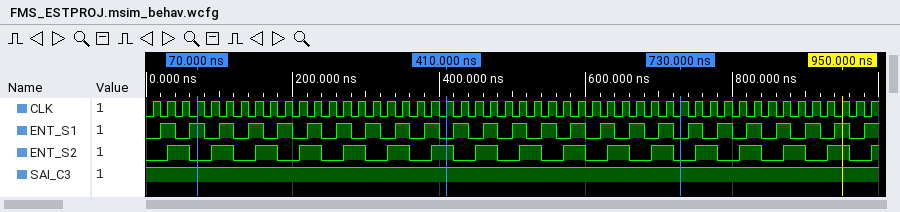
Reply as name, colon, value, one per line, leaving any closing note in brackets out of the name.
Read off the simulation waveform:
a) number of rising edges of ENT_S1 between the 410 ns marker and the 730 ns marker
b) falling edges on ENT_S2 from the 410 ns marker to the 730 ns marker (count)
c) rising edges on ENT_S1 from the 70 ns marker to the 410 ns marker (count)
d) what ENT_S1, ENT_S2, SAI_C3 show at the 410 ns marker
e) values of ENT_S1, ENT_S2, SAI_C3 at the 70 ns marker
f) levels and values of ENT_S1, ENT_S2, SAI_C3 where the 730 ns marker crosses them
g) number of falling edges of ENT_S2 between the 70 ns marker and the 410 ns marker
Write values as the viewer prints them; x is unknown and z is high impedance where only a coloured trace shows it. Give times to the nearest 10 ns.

number of rising edges of ENT_S1 between the 410 ns marker and the 730 ns marker: 8
falling edges on ENT_S2 from the 410 ns marker to the 730 ns marker: 6
rising edges on ENT_S1 from the 70 ns marker to the 410 ns marker: 8
what ENT_S1, ENT_S2, SAI_C3 show at the 410 ns marker: ENT_S1=0, ENT_S2=1, SAI_C3=1
values of ENT_S1, ENT_S2, SAI_C3 at the 70 ns marker: ENT_S1=1, ENT_S2=0, SAI_C3=1
levels and values of ENT_S1, ENT_S2, SAI_C3 where the 730 ns marker crosses them: ENT_S1=0, ENT_S2=0, SAI_C3=1
number of falling edges of ENT_S2 between the 70 ns marker and the 410 ns marker: 5
